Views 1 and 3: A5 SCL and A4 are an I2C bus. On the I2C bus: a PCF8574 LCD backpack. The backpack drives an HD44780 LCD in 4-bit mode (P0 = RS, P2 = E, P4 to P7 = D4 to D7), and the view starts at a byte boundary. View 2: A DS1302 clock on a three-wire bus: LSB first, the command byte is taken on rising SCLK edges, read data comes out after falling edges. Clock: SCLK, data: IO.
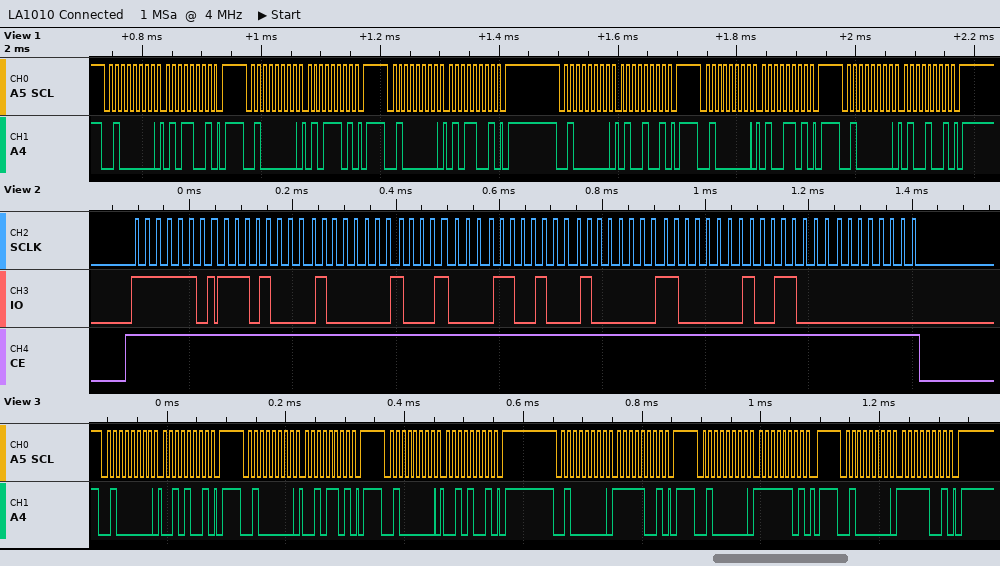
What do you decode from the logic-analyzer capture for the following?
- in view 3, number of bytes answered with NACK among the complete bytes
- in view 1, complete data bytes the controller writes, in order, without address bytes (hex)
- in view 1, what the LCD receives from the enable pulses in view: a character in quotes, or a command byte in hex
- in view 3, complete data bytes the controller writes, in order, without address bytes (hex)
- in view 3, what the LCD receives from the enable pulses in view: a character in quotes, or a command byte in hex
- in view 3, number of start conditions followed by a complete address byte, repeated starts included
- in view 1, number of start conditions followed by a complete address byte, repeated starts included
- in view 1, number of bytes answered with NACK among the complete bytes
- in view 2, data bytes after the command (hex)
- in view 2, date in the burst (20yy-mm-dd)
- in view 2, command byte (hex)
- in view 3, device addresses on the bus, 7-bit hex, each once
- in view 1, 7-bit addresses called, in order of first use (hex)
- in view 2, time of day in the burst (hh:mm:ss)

0
59 5D 59 49 4D 49
'T'
29 2D 29 F9 FD F9
'/'
6
6
0
17 02 11 26 02 03 19 00
2019-02-26
0xBF
0x20
0x20
11:02:17
